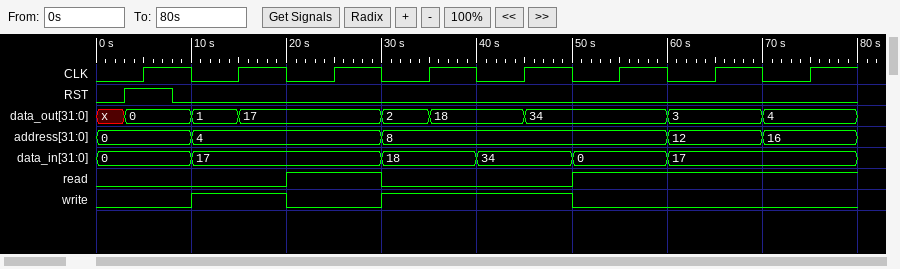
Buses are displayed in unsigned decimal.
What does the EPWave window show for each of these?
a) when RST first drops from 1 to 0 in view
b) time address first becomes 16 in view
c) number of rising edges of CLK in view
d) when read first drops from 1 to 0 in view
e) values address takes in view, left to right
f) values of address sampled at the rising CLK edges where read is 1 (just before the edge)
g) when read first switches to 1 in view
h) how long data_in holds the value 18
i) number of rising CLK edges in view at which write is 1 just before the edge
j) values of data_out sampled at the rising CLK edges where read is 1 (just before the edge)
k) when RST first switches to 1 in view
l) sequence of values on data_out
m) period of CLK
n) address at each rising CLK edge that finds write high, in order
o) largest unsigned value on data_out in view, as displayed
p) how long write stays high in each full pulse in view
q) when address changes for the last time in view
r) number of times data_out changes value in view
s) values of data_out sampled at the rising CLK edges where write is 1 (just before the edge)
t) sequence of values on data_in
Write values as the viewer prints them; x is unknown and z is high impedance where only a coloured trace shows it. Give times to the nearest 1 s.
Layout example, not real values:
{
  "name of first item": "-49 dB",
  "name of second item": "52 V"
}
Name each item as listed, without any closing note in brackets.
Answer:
{
  "when RST first drops from 1 to 0 in view": "8 s",
  "time address first becomes 16 in view": "70 s",
  "number of rising edges of CLK in view": "8",
  "when read first drops from 1 to 0 in view": "30 s",
  "values address takes in view, left to right": "0, 4, 8, 12, 16",
  "values of address sampled at the rising CLK edges where read is 1": "4, 8, 12, 16",
  "when read first switches to 1 in view": "20 s",
  "how long data_in holds the value 18": "10 s",
  "number of rising CLK edges in view at which write is 1 just before the edge": "3",
  "values of data_out sampled at the rising CLK edges where read is 1": "17, 34, 3, 4",
  "when RST first switches to 1 in view": "3 s",
  "sequence of values on data_out": "x, 0, 1, 17, 2, 18, 34, 3, 4",
  "period of CLK": "10 s",
  "address at each rising CLK edge that finds write high, in order": "4, 8, 8",
  "largest unsigned value on data_out in view, as displayed": "34",
  "how long write stays high in each full pulse in view": "10 s, 20 s",
  "when address changes for the last time in view": "70 s",
  "number of times data_out changes value in view": "8",
  "values of data_out sampled at the rising CLK edges where write is 1": "1, 2, 18",
  "sequence of values on data_in": "0, 17, 18, 34, 0, 17"
}
